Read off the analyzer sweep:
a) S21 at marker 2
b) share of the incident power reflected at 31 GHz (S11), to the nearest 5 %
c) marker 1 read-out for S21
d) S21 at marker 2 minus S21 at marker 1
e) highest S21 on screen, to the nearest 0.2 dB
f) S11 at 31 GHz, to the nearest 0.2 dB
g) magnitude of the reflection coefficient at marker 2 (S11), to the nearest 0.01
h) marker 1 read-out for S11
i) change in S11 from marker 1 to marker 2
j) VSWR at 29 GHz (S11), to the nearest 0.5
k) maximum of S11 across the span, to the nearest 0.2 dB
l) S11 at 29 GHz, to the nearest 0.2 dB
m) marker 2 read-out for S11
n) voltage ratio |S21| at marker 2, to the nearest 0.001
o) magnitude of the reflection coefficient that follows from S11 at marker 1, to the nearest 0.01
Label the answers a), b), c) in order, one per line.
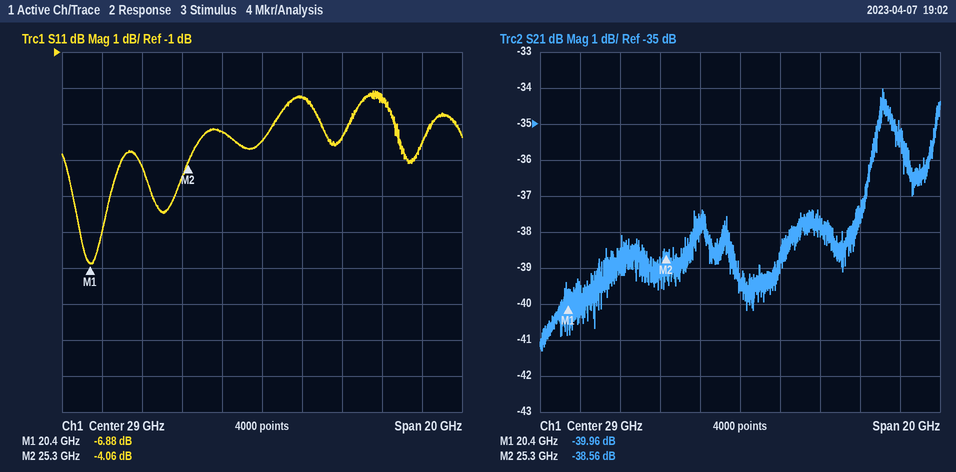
a) -38.56 dB
b) 60 %
c) -39.96 dB
d) 1.40 dB
e) -34.0 dB
f) -2.2 dB
g) 0.63
h) -6.88 dB
i) 2.82 dB
j) 5.0
k) -2.0 dB
l) -3.4 dB
m) -4.06 dB
n) 0.012
o) 0.45
